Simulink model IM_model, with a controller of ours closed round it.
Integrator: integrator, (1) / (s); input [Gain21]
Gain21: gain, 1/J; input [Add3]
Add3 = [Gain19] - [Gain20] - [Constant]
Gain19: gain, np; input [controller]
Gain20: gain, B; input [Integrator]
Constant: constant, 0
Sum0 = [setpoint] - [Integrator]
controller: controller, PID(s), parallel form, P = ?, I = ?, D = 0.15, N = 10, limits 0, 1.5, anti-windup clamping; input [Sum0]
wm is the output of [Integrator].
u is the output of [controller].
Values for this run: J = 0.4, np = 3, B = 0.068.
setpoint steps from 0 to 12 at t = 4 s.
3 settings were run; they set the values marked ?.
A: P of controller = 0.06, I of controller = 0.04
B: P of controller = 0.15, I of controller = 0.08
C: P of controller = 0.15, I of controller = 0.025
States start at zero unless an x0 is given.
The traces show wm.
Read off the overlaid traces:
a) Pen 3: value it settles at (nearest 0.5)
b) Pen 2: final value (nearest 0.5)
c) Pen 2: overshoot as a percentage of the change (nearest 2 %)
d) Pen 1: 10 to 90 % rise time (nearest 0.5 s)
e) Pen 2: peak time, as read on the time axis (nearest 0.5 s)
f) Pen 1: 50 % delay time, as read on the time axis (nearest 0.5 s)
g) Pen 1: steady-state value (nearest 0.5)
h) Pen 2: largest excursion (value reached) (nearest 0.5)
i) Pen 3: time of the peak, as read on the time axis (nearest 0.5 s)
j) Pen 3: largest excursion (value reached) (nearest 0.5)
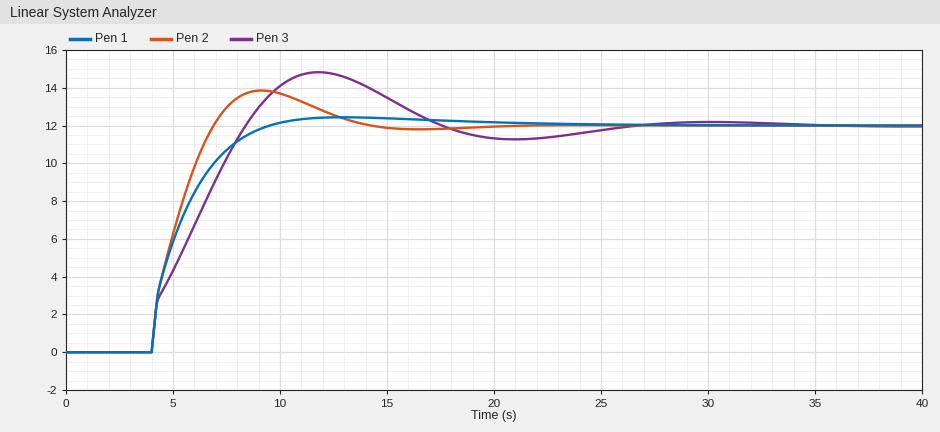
12.0
12.0
16 %
3.5 s
9.0 s
5.0 s
12.0
14.0
12.0 s
15.0
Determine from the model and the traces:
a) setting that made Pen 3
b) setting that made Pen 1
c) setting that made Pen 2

A
C
B
